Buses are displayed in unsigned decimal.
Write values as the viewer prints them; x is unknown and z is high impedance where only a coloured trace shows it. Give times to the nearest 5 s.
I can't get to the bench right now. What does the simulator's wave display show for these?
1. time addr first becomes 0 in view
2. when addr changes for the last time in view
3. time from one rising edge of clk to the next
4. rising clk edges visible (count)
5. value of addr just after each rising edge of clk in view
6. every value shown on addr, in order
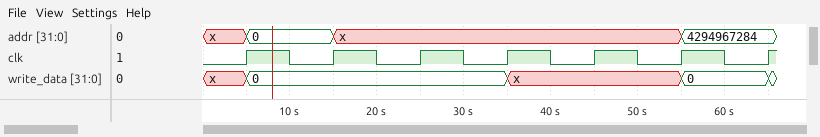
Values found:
5 s
55 s
10 s
7
0, x, x, x, x, 4294967284, 4294967284
x, 0, x, 4294967284
